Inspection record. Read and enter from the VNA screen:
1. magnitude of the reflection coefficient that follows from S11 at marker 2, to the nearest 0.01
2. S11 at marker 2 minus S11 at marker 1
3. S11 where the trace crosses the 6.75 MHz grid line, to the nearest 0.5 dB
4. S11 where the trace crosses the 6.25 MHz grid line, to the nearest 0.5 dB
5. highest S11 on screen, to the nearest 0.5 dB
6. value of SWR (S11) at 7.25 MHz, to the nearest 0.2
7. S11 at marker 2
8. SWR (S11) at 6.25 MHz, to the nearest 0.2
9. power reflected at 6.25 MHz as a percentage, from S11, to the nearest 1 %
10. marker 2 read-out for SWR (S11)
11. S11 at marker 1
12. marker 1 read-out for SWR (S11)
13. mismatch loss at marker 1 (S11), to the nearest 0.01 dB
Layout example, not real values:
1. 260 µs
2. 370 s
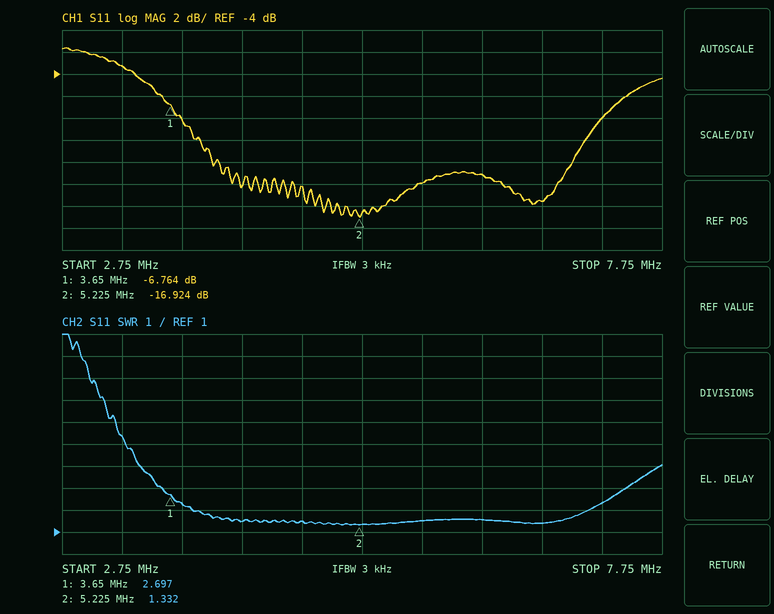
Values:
1. 0.14
2. -10.160 dB
3. -15.5 dB
4. -13.0 dB
5. -1.5 dB
6. 2.4
7. -16.924 dB
8. 1.6
9. 5 %
10. 1.332
11. -6.764 dB
12. 2.697
13. 1.03 dB
